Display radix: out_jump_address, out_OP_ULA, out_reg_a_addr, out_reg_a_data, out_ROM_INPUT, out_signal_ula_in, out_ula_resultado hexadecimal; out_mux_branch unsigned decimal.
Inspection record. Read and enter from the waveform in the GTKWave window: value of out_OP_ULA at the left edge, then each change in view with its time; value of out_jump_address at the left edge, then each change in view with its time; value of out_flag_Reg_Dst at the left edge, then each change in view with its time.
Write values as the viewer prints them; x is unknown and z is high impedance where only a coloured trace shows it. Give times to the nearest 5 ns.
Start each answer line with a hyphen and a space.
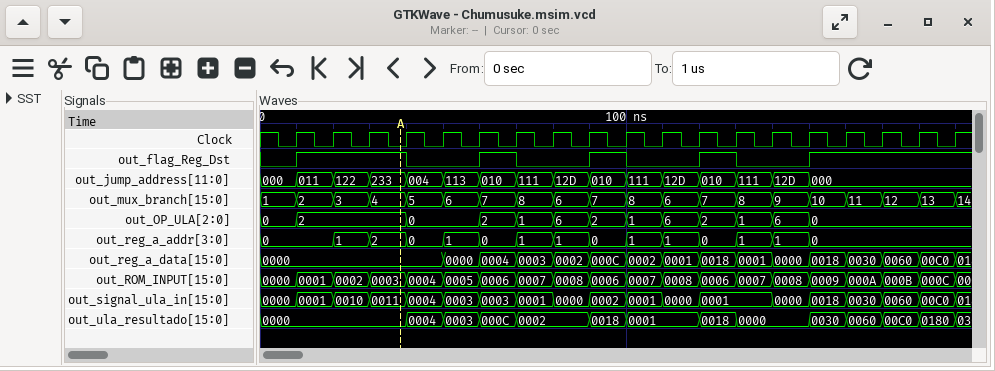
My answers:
- 0, 2 at 10 ns, 0 at 40 ns, 2 at 60 ns, 1 at 70 ns, 6 at 80 ns, 2 at 90 ns, 1 at 100 ns, 6 at 110 ns, 2 at 120 ns, 1 at 130 ns, 6 at 140 ns, 0 at 150 ns
- 000, 011 at 10 ns, 122 at 20 ns, 233 at 30 ns, 004 at 40 ns, 113 at 50 ns, 010 at 60 ns, 111 at 70 ns, 12D at 80 ns, 010 at 90 ns, 111 at 100 ns, 12D at 110 ns, 010 at 120 ns, 111 at 130 ns, 12D at 140 ns, 000 at 150 ns
- 0, 1 at 10 ns, 0 at 40 ns, 1 at 60 ns, 0 at 70 ns, 1 at 90 ns, 0 at 100 ns, 1 at 120 ns, 0 at 130 ns, 1 at 150 ns
